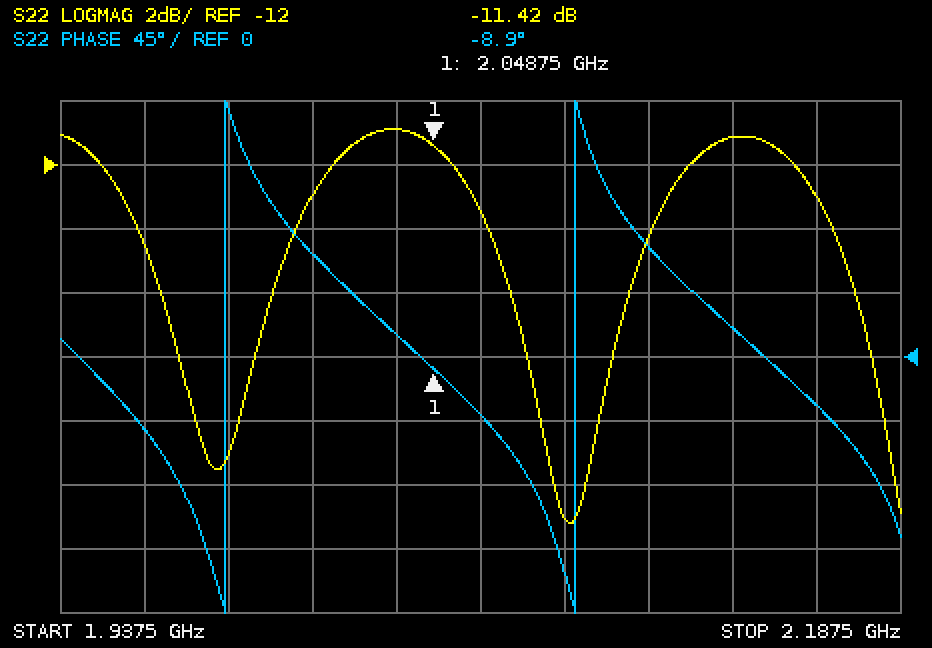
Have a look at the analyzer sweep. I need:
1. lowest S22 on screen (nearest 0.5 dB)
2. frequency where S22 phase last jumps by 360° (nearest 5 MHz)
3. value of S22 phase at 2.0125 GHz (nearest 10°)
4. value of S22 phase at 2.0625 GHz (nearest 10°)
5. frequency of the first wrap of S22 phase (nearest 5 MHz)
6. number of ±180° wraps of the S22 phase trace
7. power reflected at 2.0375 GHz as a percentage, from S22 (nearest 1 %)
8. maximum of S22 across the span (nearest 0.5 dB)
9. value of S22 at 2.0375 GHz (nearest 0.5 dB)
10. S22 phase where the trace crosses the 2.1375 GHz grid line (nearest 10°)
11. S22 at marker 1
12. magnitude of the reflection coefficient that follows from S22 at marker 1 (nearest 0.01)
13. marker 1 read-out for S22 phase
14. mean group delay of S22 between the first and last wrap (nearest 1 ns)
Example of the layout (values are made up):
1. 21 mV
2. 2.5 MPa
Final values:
1. -23.0 dB
2. 2.090 GHz
3. 70°
4. -40°
5. 1.985 GHz
6. 2
7. 8 %
8. -11.0 dB
9. -11.0 dB
10. 20°
11. -11.42 dB
12. 0.27
13. -8.9°
14. 10 ns
